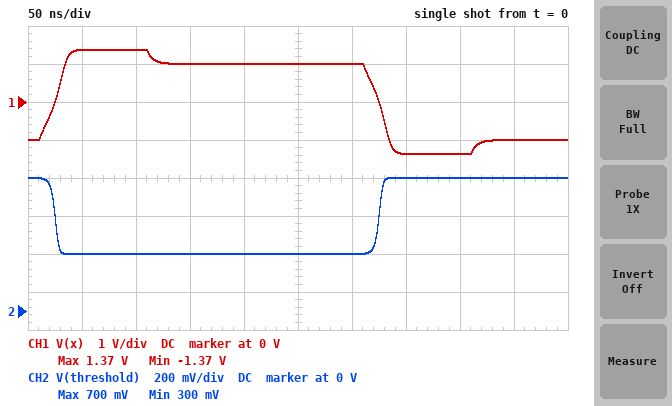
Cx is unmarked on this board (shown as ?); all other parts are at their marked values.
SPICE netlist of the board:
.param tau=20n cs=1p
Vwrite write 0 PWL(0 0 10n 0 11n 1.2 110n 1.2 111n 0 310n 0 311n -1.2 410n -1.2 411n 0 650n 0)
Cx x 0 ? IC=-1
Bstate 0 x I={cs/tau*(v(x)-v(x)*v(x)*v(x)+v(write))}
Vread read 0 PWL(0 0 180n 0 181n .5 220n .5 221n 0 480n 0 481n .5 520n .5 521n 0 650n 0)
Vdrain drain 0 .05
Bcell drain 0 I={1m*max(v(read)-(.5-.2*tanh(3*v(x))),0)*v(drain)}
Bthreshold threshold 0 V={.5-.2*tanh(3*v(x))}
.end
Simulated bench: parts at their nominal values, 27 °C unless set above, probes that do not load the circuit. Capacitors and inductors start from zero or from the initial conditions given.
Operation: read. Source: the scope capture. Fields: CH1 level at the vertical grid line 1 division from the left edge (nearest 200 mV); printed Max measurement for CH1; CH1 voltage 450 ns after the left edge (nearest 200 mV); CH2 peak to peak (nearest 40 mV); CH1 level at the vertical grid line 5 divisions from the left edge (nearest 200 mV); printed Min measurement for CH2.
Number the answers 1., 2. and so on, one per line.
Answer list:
1. 1.4 V
2. 1.37 V
3. -1.0 V
4. 400 mV
5. 1.0 V
6. 300 mV
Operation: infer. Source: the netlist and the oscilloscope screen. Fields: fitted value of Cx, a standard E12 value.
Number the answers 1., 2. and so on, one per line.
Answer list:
1. 680 fF
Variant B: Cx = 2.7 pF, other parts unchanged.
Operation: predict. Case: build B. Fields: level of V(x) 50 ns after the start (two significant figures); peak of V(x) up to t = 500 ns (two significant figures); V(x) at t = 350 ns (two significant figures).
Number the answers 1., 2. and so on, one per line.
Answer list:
1. -350 mV
2. 1.1 V
3. 350 mV
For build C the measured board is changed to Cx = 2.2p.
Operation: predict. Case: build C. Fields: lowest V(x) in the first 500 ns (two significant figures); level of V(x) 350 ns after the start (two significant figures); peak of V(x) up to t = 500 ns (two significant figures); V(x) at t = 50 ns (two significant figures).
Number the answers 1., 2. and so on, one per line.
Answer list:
1. -1.3 V
2. 190 mV
3. 1.3 V
4. -190 mV
